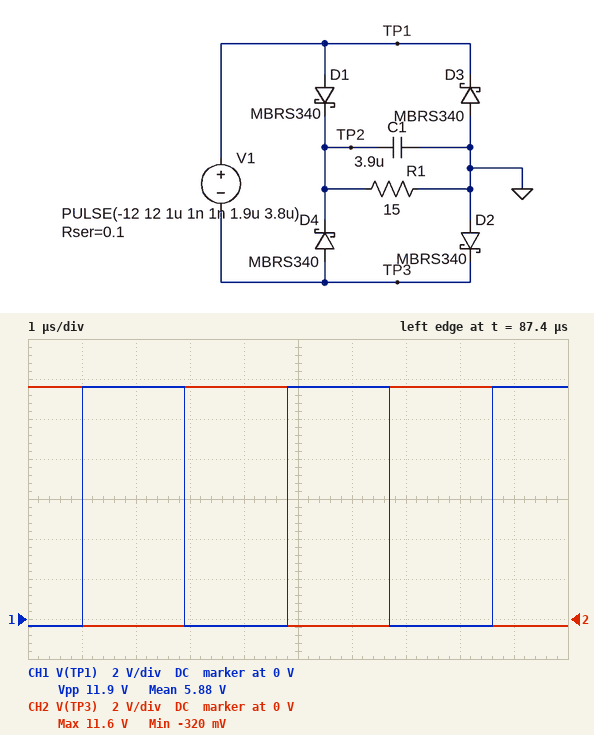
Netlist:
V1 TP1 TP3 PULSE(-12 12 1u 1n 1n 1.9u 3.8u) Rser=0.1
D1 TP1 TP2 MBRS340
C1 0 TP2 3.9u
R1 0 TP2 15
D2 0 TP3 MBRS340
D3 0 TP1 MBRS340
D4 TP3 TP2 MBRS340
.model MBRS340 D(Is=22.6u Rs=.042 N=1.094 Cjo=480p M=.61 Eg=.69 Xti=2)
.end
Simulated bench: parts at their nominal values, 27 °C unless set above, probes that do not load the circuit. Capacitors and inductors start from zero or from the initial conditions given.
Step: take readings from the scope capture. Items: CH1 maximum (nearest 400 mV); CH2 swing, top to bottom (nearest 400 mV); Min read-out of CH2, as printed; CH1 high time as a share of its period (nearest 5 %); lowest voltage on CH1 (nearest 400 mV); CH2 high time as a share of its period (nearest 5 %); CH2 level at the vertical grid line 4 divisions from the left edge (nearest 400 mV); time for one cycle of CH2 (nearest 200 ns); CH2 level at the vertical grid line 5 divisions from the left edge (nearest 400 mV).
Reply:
11.6 V
12.0 V
-320 mV
50 %
-400 mV
50 %
11.6 V
3.8 µs
-400 mV
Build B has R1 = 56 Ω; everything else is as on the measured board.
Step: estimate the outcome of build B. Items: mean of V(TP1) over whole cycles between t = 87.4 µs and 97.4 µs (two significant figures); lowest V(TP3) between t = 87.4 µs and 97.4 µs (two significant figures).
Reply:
5.7 V
-270 mV
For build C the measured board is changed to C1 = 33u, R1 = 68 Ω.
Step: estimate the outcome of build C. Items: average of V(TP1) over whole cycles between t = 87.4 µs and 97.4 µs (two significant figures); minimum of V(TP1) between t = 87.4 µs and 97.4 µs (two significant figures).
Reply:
5.7 V
-260 mV
